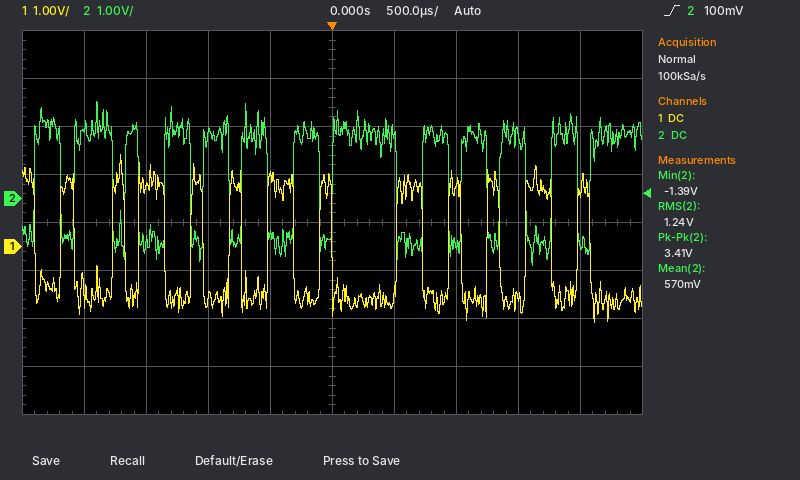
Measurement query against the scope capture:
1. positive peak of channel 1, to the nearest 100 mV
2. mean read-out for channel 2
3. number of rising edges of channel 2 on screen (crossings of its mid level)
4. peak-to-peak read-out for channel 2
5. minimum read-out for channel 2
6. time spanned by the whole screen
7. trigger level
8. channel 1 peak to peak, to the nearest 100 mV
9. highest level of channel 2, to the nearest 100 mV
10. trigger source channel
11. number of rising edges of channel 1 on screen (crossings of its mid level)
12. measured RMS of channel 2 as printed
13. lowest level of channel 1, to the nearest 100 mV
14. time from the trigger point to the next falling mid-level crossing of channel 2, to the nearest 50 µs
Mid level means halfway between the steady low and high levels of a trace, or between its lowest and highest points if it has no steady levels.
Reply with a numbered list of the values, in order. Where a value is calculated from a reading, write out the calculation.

1. 1.9 V
2. 570 mV
3. 13
4. 3.41 V
5. -1.39 V
6. 5 ms
7. 100 mV
8. 1.9 V − (-1.6 V) = 3.5 V
9. 2.0 V
10. channel 2
11. 12
12. 1.24 V
13. -1.6 V
14. 500 µs
